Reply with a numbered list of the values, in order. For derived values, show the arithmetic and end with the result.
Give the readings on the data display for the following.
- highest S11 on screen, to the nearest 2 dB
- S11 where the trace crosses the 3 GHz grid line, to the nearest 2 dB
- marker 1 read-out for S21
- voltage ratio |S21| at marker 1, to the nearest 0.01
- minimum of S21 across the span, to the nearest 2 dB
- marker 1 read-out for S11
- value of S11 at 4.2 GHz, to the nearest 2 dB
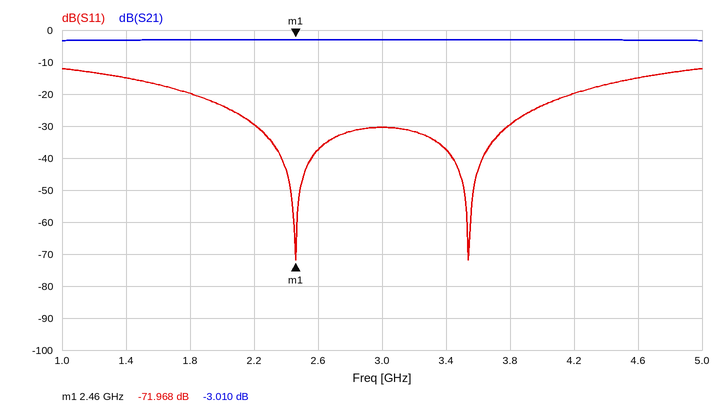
1. -12 dB
2. -30 dB
3. -3.010 dB
4. 10^(-3.01/20) ≈ 0.71
5. -4 dB
6. -71.968 dB
7. -20 dB
